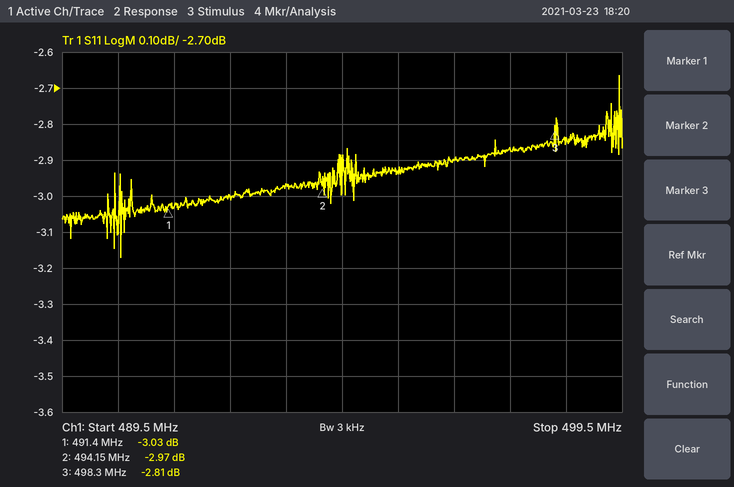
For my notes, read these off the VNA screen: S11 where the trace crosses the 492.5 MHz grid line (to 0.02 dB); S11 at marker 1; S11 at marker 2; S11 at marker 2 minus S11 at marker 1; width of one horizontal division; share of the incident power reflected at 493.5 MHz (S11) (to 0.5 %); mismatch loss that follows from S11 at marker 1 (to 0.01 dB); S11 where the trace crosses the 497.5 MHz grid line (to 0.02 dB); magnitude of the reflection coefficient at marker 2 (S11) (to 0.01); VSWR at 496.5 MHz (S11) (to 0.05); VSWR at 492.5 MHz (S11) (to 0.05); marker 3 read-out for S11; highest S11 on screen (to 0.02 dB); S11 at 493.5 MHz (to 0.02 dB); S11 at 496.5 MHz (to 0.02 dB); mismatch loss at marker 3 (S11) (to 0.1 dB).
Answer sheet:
-3.00 dB
-3.03 dB
-2.97 dB
0.06 dB
1 MHz
50.5 %
2.99 dB
-2.86 dB
0.71
6.05
5.85
-2.81 dB
-2.66 dB
-2.96 dB
-2.90 dB
3.2 dB
